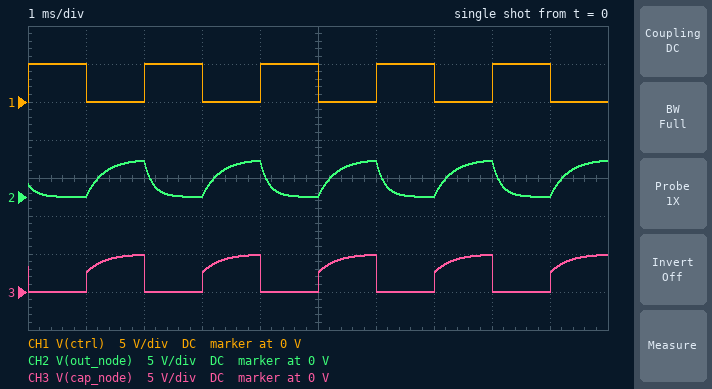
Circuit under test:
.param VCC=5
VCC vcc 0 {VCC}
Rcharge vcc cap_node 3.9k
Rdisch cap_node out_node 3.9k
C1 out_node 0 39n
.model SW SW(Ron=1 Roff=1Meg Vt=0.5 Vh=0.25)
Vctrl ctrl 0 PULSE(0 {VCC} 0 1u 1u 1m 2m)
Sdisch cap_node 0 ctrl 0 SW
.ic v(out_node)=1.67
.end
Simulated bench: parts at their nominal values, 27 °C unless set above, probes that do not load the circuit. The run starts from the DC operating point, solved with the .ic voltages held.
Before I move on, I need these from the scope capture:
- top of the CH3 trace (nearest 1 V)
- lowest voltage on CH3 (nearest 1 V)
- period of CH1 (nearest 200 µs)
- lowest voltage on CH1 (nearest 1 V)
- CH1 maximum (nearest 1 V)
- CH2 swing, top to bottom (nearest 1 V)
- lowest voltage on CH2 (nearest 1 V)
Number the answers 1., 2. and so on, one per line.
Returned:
1. 5 V
2. 0 V
3. 2.0 ms
4. 0 V
5. 5 V
6. 5 V
7. 0 V
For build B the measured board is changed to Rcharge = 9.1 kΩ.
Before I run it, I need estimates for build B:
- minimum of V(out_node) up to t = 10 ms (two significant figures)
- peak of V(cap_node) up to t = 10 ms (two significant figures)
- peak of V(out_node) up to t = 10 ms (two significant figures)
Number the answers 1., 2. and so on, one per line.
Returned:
1. 2.9 mV
2. 4.5 V
3. 4.3 V
